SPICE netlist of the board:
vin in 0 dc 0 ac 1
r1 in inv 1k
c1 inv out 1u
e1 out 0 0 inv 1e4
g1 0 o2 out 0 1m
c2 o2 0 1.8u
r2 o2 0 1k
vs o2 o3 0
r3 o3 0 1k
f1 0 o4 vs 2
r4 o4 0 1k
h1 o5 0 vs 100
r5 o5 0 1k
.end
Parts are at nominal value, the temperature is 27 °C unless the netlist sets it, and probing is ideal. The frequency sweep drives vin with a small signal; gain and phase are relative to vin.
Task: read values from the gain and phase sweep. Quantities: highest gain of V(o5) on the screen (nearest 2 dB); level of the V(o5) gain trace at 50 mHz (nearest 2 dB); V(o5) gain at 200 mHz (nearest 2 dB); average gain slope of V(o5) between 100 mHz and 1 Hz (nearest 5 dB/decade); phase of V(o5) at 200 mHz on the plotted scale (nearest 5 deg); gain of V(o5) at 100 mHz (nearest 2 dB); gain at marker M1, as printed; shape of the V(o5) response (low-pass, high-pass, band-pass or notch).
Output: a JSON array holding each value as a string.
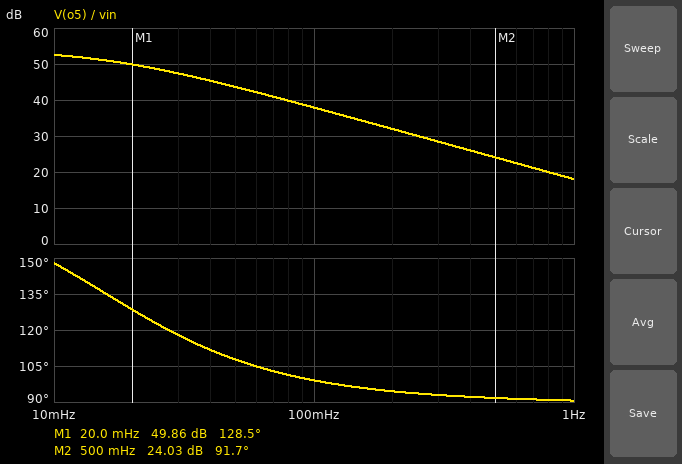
["52 dB", "44 dB", "32 dB", "-20 dB/decade", "95 deg", "38 dB", "49.86 dB", "low-pass"]
